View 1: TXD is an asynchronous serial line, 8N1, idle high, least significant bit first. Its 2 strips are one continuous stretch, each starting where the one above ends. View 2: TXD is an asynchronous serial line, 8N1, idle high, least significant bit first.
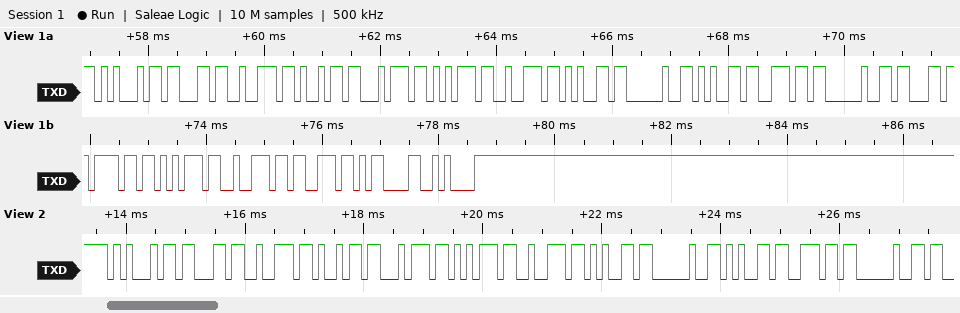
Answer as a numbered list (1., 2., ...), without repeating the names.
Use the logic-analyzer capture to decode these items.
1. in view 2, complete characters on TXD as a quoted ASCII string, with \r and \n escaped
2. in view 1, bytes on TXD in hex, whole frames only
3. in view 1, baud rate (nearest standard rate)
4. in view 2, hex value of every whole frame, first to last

1. "Ecriture en "
2. 0x45 0x63 0x72 0x69 0x74 0x75 0x72 0x65 0x20 0x65 0x6E 0x20 0x63 0x6F 0x75 0x72 0x73 0x0D 0x0A
3. 9600 baud
4. 0x45 0x63 0x72 0x69 0x74 0x75 0x72 0x65 0x20 0x65 0x6E 0x20
